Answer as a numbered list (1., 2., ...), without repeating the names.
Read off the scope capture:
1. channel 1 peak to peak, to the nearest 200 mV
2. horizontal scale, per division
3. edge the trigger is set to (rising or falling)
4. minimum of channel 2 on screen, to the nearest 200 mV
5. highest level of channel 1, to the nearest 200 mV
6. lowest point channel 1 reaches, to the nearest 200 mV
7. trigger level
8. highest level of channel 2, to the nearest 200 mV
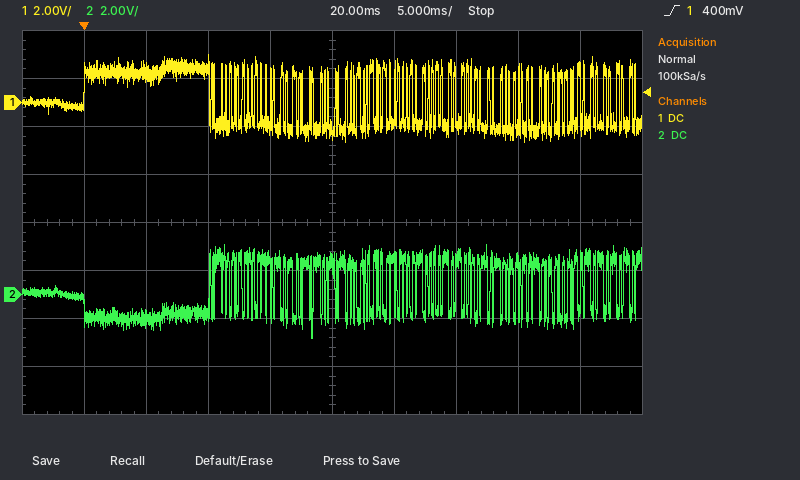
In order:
1. 3.6 V
2. 5 ms
3. rising
4. -1.8 V
5. 2.0 V
6. -1.6 V
7. 400 mV
8. 2.0 V
